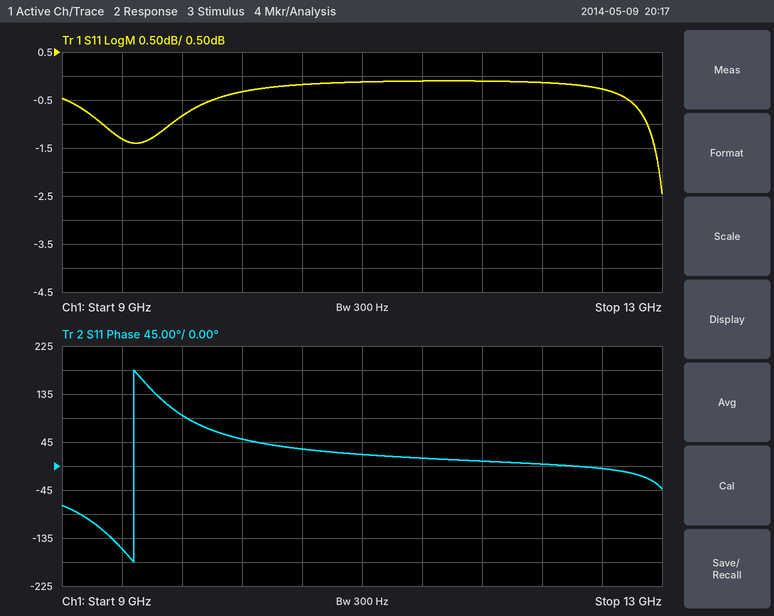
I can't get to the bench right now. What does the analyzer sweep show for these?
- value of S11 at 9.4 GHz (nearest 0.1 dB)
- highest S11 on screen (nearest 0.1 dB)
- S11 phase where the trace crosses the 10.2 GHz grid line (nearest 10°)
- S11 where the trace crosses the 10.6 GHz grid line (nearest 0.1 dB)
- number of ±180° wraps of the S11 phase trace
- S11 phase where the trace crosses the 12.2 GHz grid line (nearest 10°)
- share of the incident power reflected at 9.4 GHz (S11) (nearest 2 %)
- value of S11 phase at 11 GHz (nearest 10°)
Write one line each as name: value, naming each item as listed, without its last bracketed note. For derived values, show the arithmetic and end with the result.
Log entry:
value of S11 at 9.4 GHz: -1.3 dB
highest S11 on screen: -0.1 dB
S11 phase where the trace crosses the 10.2 GHz grid line: 50°
S11 where the trace crosses the 10.6 GHz grid line: -0.2 dB
number of ±180° wraps of the S11 phase trace: 1
S11 phase where the trace crosses the 12.2 GHz grid line: 0°
share of the incident power reflected at 9.4 GHz (S11): 10^(-1.3/10) ≈ 74 %
value of S11 phase at 11 GHz: 20°
